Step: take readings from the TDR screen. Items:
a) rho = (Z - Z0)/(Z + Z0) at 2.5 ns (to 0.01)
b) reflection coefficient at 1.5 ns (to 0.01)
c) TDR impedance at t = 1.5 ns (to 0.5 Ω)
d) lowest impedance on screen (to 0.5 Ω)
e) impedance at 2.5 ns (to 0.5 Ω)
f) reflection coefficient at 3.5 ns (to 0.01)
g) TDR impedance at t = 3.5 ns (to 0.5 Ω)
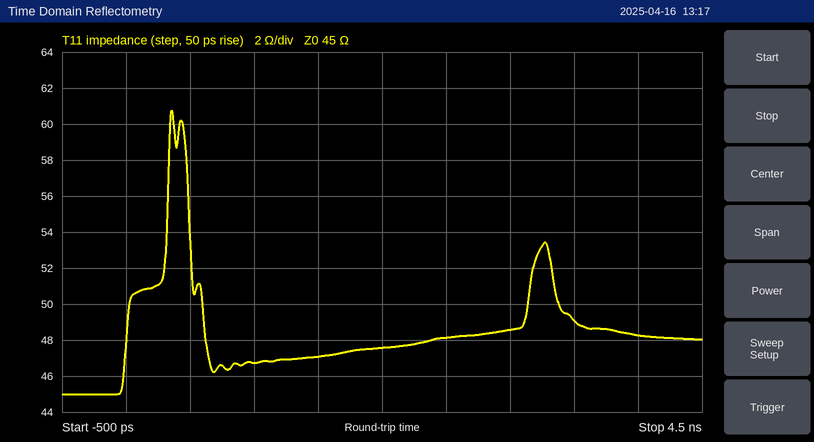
+0.03
+0.02
47.0 Ω
45.0 Ω
48.0 Ω
+0.04
49.0 Ω
